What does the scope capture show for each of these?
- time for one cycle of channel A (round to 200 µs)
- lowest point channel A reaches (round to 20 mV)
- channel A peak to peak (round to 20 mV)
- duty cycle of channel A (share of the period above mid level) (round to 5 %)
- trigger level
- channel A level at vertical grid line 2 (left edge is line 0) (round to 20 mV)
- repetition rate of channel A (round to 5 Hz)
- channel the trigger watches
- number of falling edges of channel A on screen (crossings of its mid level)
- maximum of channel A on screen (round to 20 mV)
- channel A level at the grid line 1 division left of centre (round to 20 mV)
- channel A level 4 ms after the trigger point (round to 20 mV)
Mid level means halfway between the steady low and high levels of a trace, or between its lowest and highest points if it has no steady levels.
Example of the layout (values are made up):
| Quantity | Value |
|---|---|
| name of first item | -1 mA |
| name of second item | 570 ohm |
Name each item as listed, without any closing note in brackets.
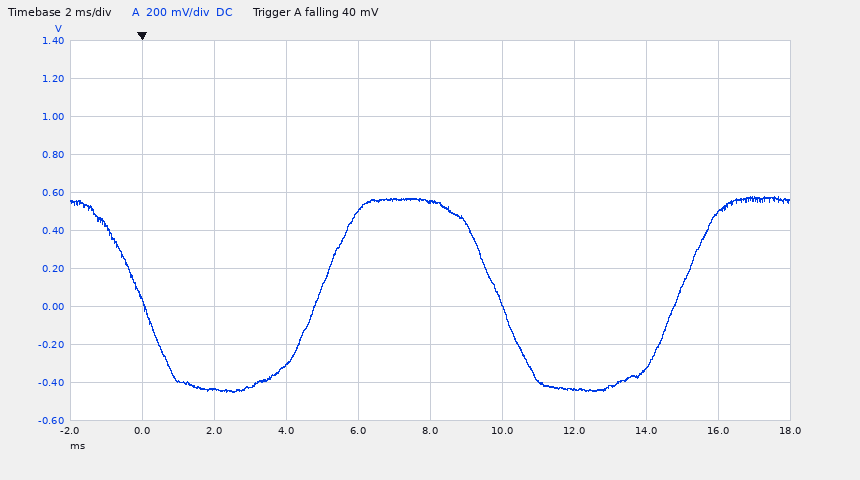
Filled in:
| Quantity | Value |
|---|---|
| time for one cycle of channel A | 10.0 ms |
| lowest point channel A reaches | -460 mV |
| channel A peak to peak | 1.04 V |
| duty cycle of channel A (share of the period above mid level) | 50 % |
| trigger level | 40 mV |
| channel A level at vertical grid line 2 (left edge is line 0) | -440 mV |
| repetition rate of channel A | 100 Hz |
| channel the trigger watches | channel A |
| number of falling edges of channel A on screen | 2 |
| maximum of channel A on screen | 580 mV |
| channel A level at the grid line 1 division left of centre | 500 mV |
| channel A level 4 ms after the trigger point | -300 mV |
